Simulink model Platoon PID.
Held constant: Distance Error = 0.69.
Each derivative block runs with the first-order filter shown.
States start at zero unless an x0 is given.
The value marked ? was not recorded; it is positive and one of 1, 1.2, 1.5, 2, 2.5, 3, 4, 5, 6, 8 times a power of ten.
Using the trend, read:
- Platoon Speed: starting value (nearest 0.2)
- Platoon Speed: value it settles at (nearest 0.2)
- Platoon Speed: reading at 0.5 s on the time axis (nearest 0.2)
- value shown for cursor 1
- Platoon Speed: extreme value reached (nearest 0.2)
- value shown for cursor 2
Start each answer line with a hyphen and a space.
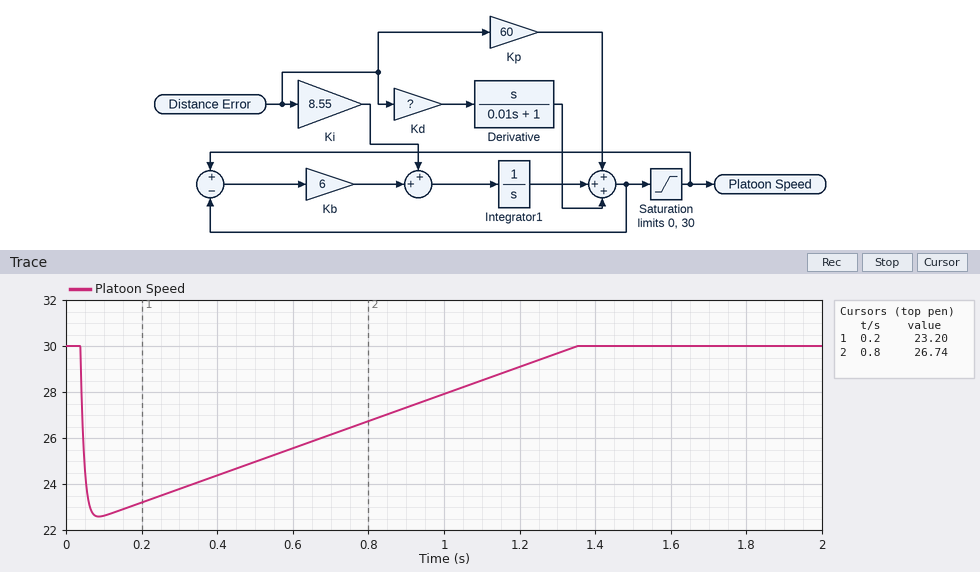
- 30.0
- 30.0
- 25.0
- 23.20
- 22.6
- 26.74
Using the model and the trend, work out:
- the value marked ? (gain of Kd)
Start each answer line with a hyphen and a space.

- 5
